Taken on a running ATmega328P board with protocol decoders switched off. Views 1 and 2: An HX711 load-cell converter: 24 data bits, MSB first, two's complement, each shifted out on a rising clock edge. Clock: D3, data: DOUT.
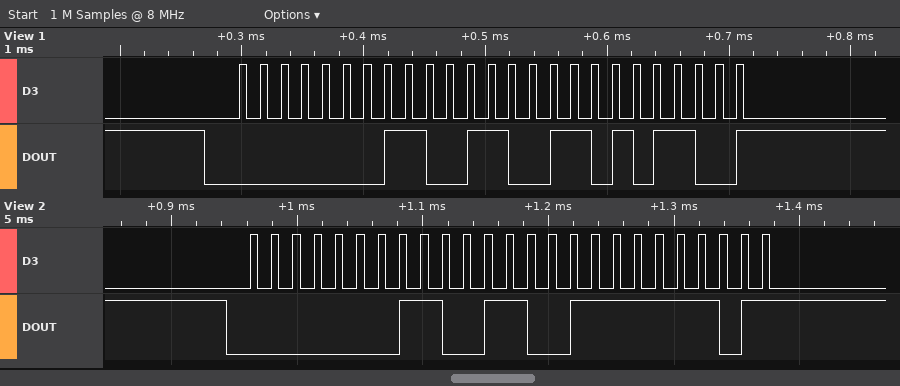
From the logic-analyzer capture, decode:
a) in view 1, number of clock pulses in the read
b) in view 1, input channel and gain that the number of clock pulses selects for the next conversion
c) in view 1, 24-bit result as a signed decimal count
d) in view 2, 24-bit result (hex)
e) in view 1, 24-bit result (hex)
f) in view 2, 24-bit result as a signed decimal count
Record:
25
channel A, gain 128
104876
0x0199FD
0x0199AC
104957
